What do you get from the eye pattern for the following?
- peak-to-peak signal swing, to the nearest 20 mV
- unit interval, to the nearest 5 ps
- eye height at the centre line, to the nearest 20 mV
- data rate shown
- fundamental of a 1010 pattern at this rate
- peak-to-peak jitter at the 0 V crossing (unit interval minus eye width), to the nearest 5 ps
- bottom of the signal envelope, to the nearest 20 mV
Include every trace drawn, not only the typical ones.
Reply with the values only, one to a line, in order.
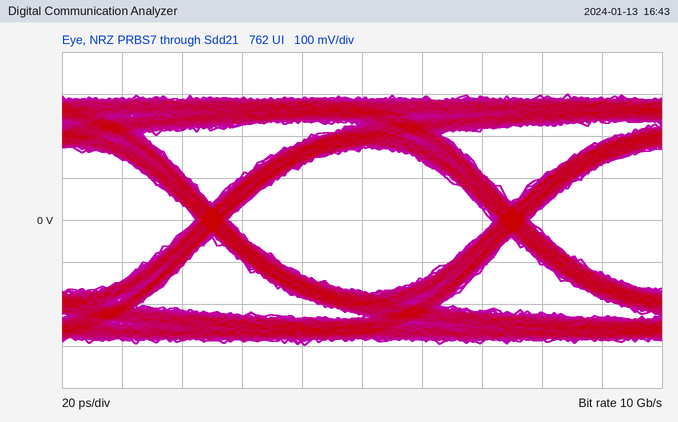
600 mV
100 ps
340 mV
10 Gb/s
5 GHz
10 ps
-300 mV
